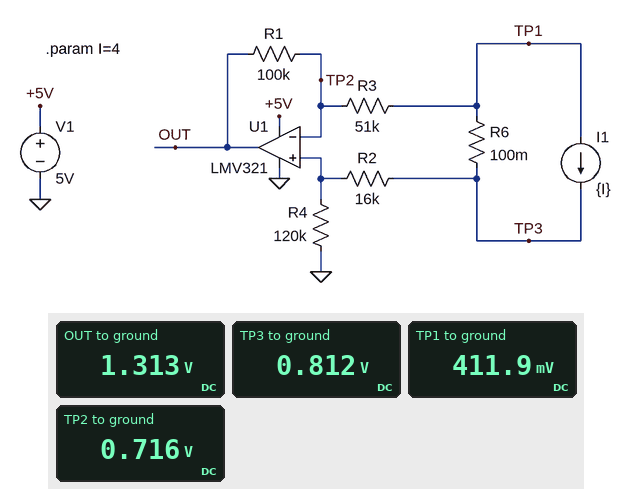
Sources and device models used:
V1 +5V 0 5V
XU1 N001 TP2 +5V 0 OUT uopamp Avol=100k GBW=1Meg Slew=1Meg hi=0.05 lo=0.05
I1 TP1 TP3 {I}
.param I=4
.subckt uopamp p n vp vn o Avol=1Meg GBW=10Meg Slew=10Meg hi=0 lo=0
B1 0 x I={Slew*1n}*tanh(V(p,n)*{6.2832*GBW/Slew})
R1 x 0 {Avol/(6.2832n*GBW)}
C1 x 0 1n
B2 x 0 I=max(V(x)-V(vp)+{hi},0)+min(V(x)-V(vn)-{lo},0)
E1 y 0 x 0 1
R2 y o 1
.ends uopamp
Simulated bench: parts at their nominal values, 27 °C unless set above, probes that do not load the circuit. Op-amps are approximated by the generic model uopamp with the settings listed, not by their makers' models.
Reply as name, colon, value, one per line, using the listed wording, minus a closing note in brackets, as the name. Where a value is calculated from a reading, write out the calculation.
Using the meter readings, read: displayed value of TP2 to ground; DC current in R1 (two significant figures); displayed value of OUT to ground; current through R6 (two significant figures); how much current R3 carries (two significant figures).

displayed value of TP2 to ground: 0.716 V
DC current in R1: (1.313 V - 716 mV) / 100 kΩ = 6.0 µA
displayed value of OUT to ground: 1.313 V
current through R6: (812 mV - 411.9 mV) / 100 mΩ = 4.0 A
how much current R3 carries: (716 mV - 411.9 mV) / 51 kΩ = 6.0 µA
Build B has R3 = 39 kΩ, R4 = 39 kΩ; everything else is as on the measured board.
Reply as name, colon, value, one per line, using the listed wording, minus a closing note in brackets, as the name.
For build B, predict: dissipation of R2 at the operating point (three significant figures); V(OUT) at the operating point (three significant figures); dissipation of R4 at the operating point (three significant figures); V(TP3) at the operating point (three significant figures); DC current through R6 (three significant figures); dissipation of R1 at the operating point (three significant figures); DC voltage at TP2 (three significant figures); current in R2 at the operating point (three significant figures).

dissipation of R2 at the operating point: 846 nW
V(OUT) at the operating point: 1.01 V
dissipation of R4 at the operating point: 2.06 µW
V(TP3) at the operating point: 400 mV
DC current through R6: 4.00 A
dissipation of R1 at the operating point: 5.29 µW
DC voltage at TP2: 284 mV
current in R2 at the operating point: 7.27 µA
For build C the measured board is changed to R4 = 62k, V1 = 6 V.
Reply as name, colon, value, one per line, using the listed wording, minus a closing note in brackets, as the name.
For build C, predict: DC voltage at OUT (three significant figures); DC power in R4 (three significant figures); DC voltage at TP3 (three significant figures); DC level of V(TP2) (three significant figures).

DC voltage at OUT: 967 mV
DC power in R4: 2.21 µW
DC voltage at TP3: 466 mV
DC level of V(TP2): 370 mV
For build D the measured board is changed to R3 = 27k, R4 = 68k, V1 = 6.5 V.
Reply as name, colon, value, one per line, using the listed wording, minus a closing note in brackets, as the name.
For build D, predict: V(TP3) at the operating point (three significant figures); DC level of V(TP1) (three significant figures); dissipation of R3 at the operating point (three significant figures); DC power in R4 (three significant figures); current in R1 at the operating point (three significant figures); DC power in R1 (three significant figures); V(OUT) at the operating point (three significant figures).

V(TP3) at the operating point: 781 mV
DC level of V(TP1): 381 mV
dissipation of R3 at the operating point: 2.34 µW
DC power in R4: 5.88 µW
current in R1 at the operating point: 9.30 µA
DC power in R1: 8.65 µW
V(OUT) at the operating point: 1.56 V
